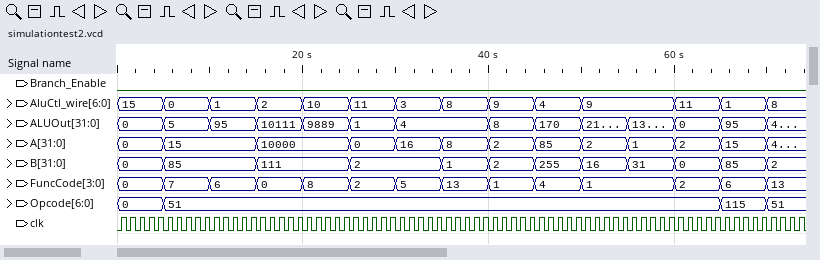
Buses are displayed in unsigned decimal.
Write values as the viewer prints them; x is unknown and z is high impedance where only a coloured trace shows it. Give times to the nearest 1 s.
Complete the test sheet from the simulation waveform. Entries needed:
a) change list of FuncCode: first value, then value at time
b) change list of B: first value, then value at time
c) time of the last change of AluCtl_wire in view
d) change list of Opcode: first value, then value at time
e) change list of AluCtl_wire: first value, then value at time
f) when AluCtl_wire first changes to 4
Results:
0, 7 at 5 s, 6 at 10 s, 0 at 15 s, 8 at 20 s, 2 at 25 s, 5 at 30 s, 13 at 35 s, 1 at 40 s, 4 at 45 s, 1 at 50 s, 2 at 60 s, 6 at 65 s, 13 at 70 s
0, 85 at 5 s, 111 at 15 s, 2 at 25 s, 1 at 35 s, 2 at 40 s, 255 at 45 s, 16 at 50 s, 31 at 55 s, 0 at 60 s, 85 at 65 s, 2 at 70 s
70 s
0, 51 at 5 s, 115 at 65 s, 51 at 70 s
15, 0 at 5 s, 1 at 10 s, 2 at 15 s, 10 at 20 s, 11 at 25 s, 3 at 30 s, 8 at 35 s, 9 at 40 s, 4 at 45 s, 9 at 50 s, 11 at 60 s, 1 at 65 s, 8 at 70 s
45 s
